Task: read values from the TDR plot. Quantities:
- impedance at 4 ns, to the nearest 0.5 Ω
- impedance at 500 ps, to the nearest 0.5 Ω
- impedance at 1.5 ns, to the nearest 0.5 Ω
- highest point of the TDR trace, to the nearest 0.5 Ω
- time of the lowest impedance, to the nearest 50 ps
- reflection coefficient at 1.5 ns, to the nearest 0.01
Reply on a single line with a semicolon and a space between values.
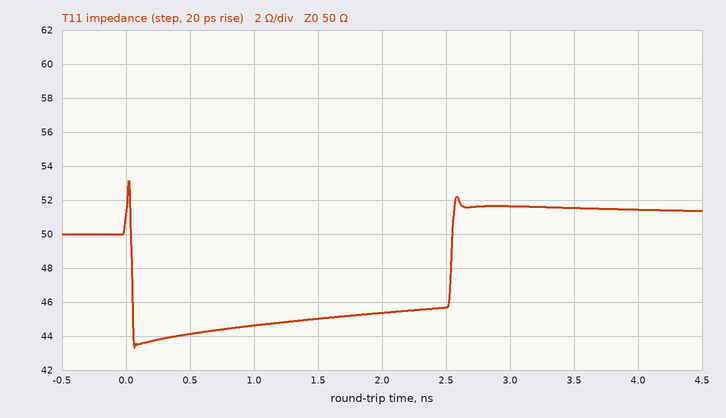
51.5 Ω; 44.0 Ω; 45.0 Ω; 53.0 Ω; 50 ps; -0.05
